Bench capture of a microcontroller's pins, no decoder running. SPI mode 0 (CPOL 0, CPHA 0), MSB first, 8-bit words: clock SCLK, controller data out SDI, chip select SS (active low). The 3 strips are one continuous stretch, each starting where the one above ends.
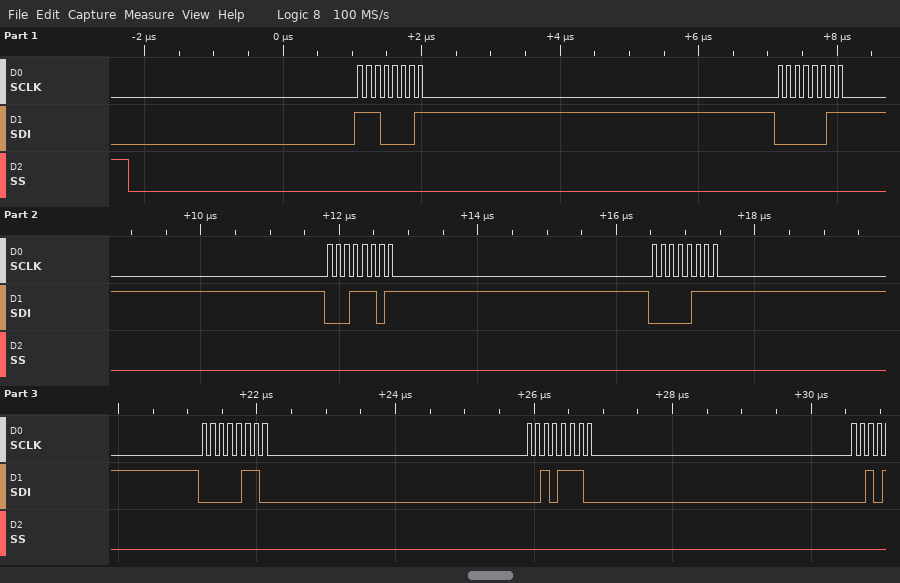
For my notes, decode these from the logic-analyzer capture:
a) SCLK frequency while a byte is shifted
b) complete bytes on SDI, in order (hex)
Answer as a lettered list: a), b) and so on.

a) 8 MHz
b) 0xE1 0x03 0x1D 0x07 0x06 0x2E
